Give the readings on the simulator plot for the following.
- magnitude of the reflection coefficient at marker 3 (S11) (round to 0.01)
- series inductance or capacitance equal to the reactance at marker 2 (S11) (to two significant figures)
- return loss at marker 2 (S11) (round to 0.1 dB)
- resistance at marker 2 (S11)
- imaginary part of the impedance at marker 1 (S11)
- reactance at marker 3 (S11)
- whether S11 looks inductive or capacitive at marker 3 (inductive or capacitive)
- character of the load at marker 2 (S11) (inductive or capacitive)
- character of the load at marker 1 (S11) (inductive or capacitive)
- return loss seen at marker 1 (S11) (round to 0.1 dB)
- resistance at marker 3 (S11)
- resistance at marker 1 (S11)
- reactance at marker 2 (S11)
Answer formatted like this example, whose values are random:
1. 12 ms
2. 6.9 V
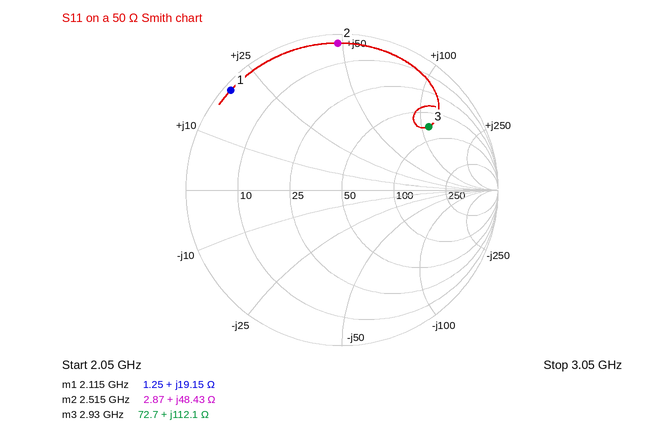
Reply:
1. 0.69
2. 3.1 nH
3. 0.5 dB
4. 2.87 Ω
5. +19.15 Ω
6. +112.1 Ω
7. inductive
8. inductive
9. inductive
10. 0.4 dB
11. 72.7 Ω
12. 1.25 Ω
13. +48.43 Ω
